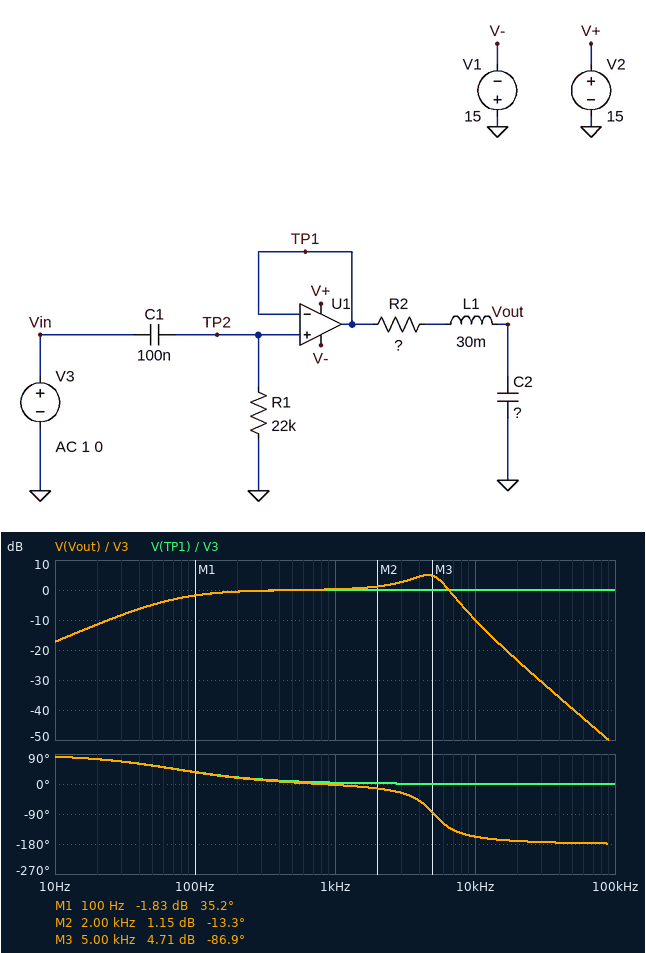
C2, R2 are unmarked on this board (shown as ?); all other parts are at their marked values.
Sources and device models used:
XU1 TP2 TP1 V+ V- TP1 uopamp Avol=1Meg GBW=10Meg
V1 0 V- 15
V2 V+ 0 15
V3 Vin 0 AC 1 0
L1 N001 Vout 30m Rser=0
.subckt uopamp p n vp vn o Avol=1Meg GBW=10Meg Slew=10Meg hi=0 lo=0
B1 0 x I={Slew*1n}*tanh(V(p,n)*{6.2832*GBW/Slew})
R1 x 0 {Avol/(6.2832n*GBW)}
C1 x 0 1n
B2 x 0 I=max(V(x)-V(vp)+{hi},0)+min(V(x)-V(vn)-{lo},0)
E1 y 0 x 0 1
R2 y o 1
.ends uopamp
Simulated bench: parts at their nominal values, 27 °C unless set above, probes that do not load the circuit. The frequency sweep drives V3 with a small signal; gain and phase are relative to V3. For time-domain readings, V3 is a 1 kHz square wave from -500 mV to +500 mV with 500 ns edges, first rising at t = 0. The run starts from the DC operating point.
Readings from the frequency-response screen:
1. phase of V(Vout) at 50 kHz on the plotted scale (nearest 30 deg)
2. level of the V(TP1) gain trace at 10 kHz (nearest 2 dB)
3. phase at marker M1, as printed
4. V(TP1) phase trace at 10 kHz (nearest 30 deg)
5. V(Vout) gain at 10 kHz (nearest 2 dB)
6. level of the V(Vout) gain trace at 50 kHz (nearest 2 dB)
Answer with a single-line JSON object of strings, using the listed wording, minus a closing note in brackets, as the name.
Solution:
{"phase of V(Vout) at 50 kHz on the plotted scale": "-180 deg", "level of the V(TP1) gain trace at 10 kHz": "0 dB", "phase at marker M1, as printed": "35.2 deg", "V(TP1) phase trace at 10 kHz": "0 deg", "V(Vout) gain at 10 kHz": "-10 dB", "level of the V(Vout) gain trace at 50 kHz": "-40 dB"}
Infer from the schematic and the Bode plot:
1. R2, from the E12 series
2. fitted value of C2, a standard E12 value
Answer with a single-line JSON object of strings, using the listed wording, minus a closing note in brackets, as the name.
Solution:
{"R2, from the E12 series": "560 Ω", "fitted value of C2, a standard E12 value": "33 nF"}
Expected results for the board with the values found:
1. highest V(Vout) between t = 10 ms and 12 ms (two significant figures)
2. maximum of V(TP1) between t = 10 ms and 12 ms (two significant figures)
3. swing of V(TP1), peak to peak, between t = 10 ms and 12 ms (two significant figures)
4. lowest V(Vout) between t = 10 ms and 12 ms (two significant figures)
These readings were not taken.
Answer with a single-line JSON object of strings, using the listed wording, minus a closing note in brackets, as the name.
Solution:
{"highest V(Vout) between t = 10 ms and 12 ms": "930 mV", "maximum of V(TP1) between t = 10 ms and 12 ms": "560 mV", "swing of V(TP1), peak to peak, between t = 10 ms and 12 ms": "1.1 V", "lowest V(Vout) between t = 10 ms and 12 ms": "-920 mV"}
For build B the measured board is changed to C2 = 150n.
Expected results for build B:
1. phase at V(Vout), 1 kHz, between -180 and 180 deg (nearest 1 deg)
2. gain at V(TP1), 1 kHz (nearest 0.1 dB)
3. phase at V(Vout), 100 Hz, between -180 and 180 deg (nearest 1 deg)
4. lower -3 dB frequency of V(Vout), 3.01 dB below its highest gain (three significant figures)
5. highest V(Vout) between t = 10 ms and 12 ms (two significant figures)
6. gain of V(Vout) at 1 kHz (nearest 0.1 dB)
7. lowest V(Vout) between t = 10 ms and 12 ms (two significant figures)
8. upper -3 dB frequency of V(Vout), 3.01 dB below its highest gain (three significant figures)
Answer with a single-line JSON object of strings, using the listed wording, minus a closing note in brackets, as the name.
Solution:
{"phase at V(Vout), 1 kHz, between -180 and 180 deg": "-29 deg", "gain at V(TP1), 1 kHz": "0 dB", "phase at V(Vout), 100 Hz, between -180 and 180 deg": "33 deg", "lower -3 dB frequency of V(Vout), 3.01 dB below its highest gain": "75.6 Hz", "highest V(Vout) between t = 10 ms and 12 ms": "600 mV", "gain of V(Vout) at 1 kHz": "0.2 dB", "lowest V(Vout) between t = 10 ms and 12 ms": "-590 mV", "upper -3 dB frequency of V(Vout), 3.01 dB below its highest gain": "2.59 kHz"}
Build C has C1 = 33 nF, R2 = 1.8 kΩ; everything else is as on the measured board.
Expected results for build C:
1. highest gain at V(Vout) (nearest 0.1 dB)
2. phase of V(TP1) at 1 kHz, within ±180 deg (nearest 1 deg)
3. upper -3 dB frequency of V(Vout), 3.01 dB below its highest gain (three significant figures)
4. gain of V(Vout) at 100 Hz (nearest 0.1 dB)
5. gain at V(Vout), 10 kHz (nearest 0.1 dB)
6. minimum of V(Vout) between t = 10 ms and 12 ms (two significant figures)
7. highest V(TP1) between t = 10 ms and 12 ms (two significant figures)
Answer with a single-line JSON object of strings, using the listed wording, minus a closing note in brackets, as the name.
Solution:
{"highest gain at V(Vout)": "-0.5 dB", "phase of V(TP1) at 1 kHz, within ±180 deg": "12 deg", "upper -3 dB frequency of V(Vout), 3.01 dB below its highest gain": "3.82 kHz", "gain of V(Vout) at 100 Hz": "-7.6 dB", "gain at V(Vout), 10 kHz": "-13.5 dB", "minimum of V(Vout) between t = 10 ms and 12 ms": "-560 mV", "highest V(TP1) between t = 10 ms and 12 ms": "670 mV"}
